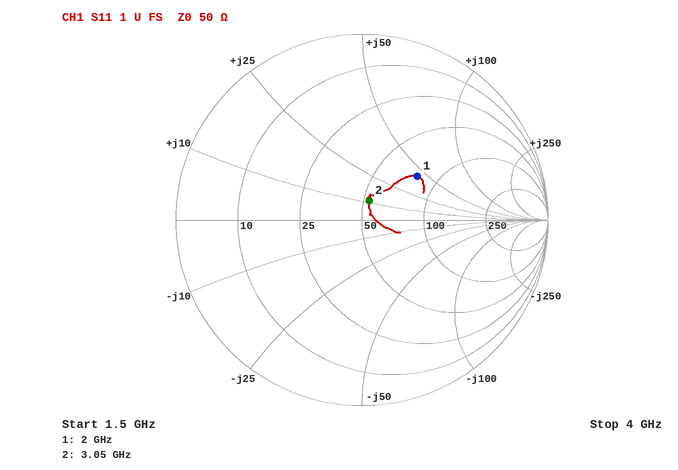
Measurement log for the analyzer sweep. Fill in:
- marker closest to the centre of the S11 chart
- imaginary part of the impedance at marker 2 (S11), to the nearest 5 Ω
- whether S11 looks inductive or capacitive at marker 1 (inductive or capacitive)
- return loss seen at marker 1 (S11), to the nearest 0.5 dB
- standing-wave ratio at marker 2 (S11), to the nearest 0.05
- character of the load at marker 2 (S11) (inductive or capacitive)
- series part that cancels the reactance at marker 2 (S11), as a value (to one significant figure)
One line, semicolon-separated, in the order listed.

marker 2; +10 Ω; inductive; 8.5 dB; 1.25; inductive; 5 pF
